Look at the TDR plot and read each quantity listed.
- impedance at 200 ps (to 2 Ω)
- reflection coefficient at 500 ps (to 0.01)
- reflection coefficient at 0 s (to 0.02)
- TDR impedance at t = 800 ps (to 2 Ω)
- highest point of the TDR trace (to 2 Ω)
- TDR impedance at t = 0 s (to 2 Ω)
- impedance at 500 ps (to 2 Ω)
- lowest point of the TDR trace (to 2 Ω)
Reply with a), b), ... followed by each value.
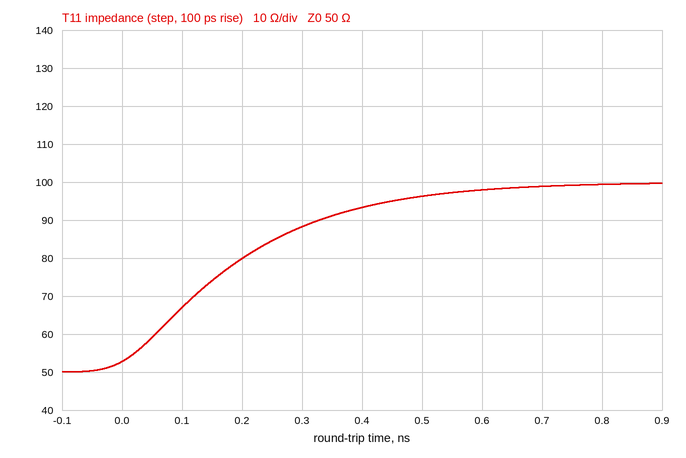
a) 80 Ω
b) +0.32
c) +0.02
d) 100 Ω
e) 100 Ω
f) 52 Ω
g) 96 Ω
h) 50 Ω
